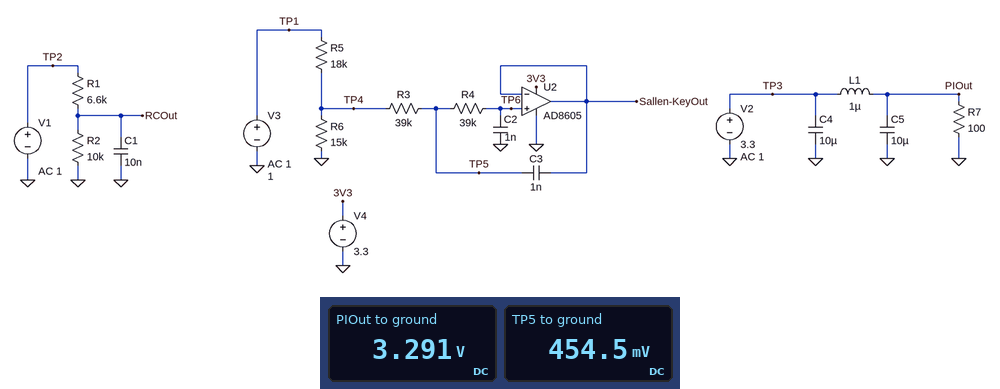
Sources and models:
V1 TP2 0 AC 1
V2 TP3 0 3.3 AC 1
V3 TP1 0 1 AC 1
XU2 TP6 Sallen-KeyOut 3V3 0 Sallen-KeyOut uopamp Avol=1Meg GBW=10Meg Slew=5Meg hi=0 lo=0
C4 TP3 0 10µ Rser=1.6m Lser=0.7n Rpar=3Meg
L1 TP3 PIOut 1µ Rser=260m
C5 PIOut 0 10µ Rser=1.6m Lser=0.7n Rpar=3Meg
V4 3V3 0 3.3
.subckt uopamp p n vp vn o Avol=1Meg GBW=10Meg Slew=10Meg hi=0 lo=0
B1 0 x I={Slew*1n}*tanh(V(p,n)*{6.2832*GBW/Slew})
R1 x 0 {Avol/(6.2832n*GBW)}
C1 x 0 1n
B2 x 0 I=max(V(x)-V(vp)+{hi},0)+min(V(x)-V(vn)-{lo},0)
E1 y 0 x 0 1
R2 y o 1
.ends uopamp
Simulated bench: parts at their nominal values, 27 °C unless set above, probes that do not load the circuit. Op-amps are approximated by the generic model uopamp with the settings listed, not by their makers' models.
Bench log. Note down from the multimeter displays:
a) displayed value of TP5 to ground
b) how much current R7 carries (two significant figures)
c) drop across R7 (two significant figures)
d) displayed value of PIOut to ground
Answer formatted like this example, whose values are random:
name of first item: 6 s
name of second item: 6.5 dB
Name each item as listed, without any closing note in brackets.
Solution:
displayed value of TP5 to ground: 454.5 mV
how much current R7 carries: 33 mA
drop across R7: 3.3 V
displayed value of PIOut to ground: 3.291 V
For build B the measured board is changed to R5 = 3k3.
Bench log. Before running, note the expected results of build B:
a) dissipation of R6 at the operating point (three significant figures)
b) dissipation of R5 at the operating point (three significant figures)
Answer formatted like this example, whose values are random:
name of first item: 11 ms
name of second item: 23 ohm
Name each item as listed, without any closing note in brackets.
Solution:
dissipation of R6 at the operating point: 44.8 µW
dissipation of R5 at the operating point: 9.85 µW
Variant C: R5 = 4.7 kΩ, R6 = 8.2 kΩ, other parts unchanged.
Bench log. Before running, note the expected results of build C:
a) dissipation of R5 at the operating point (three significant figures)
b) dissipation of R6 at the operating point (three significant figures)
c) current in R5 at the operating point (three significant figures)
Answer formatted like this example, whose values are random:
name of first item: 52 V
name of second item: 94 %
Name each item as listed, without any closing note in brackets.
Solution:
dissipation of R5 at the operating point: 28.2 µW
dissipation of R6 at the operating point: 49.3 µW
current in R5 at the operating point: 77.5 µA
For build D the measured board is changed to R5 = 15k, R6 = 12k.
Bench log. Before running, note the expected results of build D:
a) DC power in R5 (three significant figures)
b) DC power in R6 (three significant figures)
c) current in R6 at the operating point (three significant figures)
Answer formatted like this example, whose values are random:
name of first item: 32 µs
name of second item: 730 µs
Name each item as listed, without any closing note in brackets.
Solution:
DC power in R5: 20.6 µW
DC power in R6: 16.5 µW
current in R6 at the operating point: 37.0 µA
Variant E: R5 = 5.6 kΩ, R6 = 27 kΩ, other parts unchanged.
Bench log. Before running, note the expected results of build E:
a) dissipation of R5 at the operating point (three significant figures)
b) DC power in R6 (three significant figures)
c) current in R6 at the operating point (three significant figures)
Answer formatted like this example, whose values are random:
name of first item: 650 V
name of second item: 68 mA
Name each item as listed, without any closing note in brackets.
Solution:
dissipation of R5 at the operating point: 5.27 µW
DC power in R6: 25.4 µW
current in R6 at the operating point: 30.7 µA
